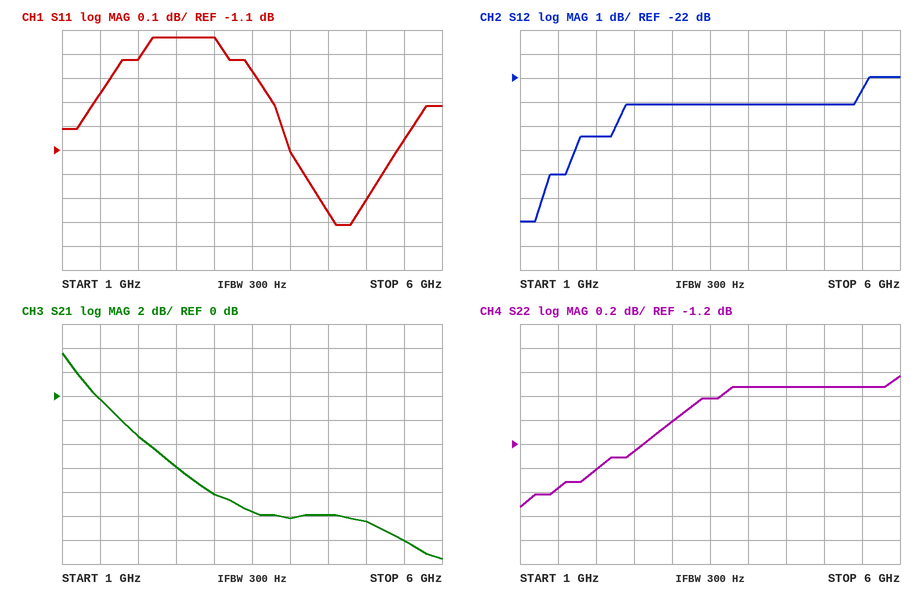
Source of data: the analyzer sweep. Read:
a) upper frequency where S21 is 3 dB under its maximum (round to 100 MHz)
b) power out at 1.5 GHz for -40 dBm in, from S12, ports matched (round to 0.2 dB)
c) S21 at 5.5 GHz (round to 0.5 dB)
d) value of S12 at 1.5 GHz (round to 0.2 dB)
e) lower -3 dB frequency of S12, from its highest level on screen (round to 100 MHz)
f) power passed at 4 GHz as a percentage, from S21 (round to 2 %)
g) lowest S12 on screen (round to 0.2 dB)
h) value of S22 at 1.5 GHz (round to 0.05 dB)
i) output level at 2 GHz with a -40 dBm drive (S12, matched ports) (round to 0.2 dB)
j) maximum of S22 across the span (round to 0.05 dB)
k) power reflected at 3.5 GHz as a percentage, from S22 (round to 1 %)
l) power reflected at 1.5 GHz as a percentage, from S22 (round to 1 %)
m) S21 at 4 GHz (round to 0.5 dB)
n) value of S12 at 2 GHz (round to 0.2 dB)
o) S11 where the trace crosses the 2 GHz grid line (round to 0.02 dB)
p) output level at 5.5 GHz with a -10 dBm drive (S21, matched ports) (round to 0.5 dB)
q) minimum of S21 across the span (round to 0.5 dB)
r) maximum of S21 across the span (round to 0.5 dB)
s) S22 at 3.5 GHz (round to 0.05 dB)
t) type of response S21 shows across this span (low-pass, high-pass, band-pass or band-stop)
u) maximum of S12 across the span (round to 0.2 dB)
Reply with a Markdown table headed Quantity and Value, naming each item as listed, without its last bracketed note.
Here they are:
| Quantity | Value |
|---|---|
| upper frequency where S21 is 3 dB under its maximum | 1.4 GHz |
| power out at 1.5 GHz for -40 dBm in, from S12, ports matched | -66.0 dBm |
| S21 at 5.5 GHz | -12.0 dB |
| value of S12 at 1.5 GHz | -26.0 dB |
| lower -3 dB frequency of S12, from its highest level on screen | 1.7 GHz |
| power passed at 4 GHz as a percentage, from S21 | 10 % |
| lowest S12 on screen | -28.0 dB |
| value of S22 at 1.5 GHz | -1.55 dB |
| output level at 2 GHz with a -40 dBm drive (S12, matched ports) | -64.4 dBm |
| maximum of S22 across the span | -0.65 dB |
| power reflected at 3.5 GHz as a percentage, from S22 | 83 % |
| power reflected at 1.5 GHz as a percentage, from S22 | 70 % |
| S21 at 4 GHz | -10.0 dB |
| value of S12 at 2 GHz | -24.4 dB |
| S11 where the trace crosses the 2 GHz grid line | -0.72 dB |
| output level at 5.5 GHz with a -10 dBm drive (S21, matched ports) | -22.0 dBm |
| minimum of S21 across the span | -13.5 dB |
| maximum of S21 across the span | 3.5 dB |
| S22 at 3.5 GHz | -0.80 dB |
| type of response S21 shows across this span | low-pass |
| maximum of S12 across the span | -22.0 dB |
